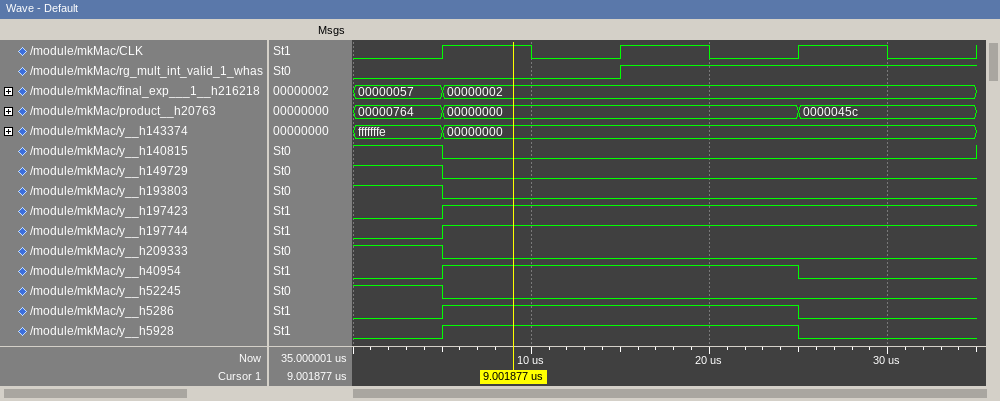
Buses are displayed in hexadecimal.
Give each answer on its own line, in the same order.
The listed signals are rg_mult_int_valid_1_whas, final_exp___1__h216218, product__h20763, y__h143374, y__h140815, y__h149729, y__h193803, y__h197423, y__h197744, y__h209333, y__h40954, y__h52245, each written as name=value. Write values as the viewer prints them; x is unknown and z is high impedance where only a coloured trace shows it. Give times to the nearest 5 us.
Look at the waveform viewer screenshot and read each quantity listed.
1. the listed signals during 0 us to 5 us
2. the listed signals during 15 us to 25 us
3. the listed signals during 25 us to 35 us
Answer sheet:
rg_mult_int_valid_1_whas=0, final_exp___1__h216218=00000057, product__h20763=00000764, y__h143374=fffffffe, y__h140815=1, y__h149729=1, y__h193803=1, y__h197423=0, y__h197744=0, y__h209333=1, y__h40954=0, y__h52245=1
rg_mult_int_valid_1_whas=1, final_exp___1__h216218=00000002, product__h20763=00000000, y__h143374=00000000, y__h140815=0, y__h149729=0, y__h193803=0, y__h197423=1, y__h197744=1, y__h209333=0, y__h40954=1, y__h52245=0
rg_mult_int_valid_1_whas=1, final_exp___1__h216218=00000002, product__h20763=0000045c, y__h143374=00000000, y__h140815=0, y__h149729=0, y__h193803=0, y__h197423=1, y__h197744=1, y__h209333=0, y__h40954=0, y__h52245=0
